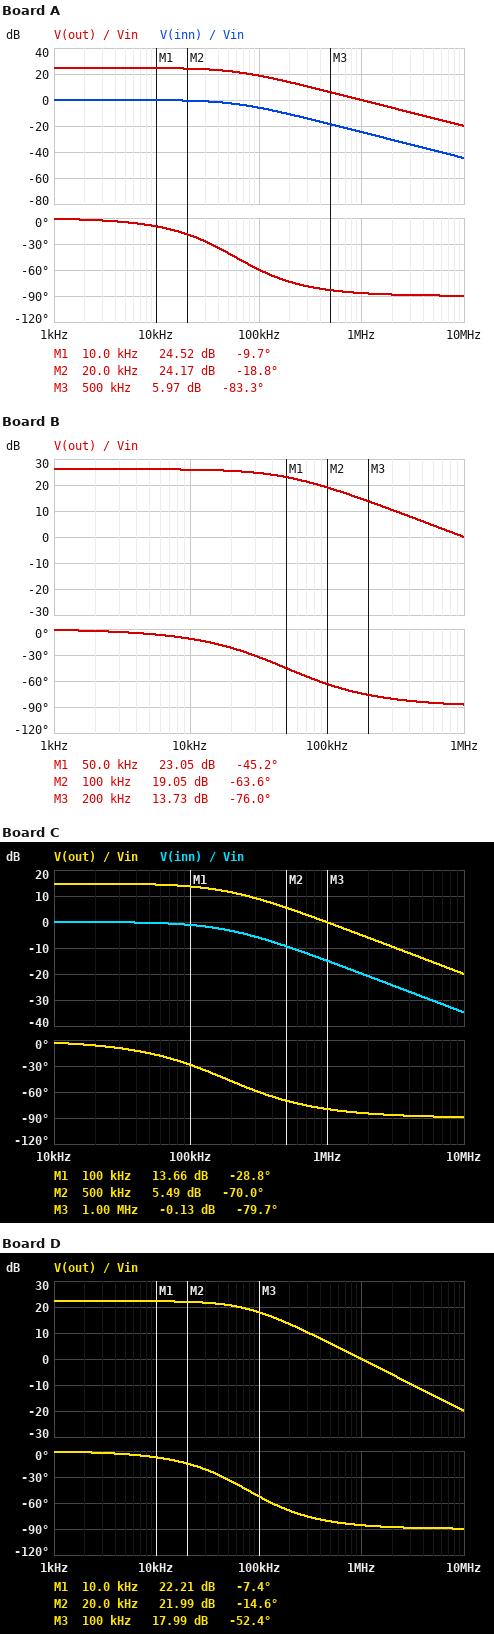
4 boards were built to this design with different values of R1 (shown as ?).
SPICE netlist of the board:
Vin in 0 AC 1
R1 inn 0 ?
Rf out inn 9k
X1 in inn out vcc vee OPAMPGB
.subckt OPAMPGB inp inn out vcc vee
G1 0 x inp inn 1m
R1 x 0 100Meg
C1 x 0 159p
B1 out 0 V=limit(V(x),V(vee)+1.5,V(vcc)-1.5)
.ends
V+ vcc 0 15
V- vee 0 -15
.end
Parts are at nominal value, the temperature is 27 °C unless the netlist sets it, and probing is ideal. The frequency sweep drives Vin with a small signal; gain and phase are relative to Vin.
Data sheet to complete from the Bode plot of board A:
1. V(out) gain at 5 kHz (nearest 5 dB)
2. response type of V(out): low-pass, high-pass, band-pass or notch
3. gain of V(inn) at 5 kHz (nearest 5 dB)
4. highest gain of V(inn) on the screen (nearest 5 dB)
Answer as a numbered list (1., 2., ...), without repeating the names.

1. 25 dB
2. low-pass
3. 0 dB
4. 0 dB
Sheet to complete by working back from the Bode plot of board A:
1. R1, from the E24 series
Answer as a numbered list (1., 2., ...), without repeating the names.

1. 560 Ω
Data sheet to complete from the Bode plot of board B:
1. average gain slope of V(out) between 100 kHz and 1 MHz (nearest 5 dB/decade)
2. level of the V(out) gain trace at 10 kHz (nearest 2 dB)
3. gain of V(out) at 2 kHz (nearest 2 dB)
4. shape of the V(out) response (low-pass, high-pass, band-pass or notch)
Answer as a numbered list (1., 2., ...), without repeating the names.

1. -20 dB/decade
2. 26 dB
3. 26 dB
4. low-pass
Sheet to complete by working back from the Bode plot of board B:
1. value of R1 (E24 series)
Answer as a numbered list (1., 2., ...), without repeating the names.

1. 470 Ω
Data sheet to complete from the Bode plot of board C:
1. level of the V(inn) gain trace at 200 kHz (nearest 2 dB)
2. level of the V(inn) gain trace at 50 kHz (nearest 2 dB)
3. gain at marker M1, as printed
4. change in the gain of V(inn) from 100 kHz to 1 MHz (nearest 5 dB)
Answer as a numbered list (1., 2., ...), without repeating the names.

1. -4 dB
2. 0 dB
3. 13.66 dB
4. -15 dB
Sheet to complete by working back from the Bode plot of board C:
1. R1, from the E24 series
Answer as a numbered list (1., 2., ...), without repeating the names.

1. 2 kΩ
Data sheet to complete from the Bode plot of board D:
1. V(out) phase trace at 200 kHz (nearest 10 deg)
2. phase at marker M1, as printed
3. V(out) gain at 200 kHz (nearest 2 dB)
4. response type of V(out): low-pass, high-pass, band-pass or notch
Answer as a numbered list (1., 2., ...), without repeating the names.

1. -70 deg
2. -7.4 deg
3. 14 dB
4. low-pass
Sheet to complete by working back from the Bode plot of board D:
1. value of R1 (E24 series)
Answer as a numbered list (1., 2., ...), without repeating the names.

1. 750 Ω
